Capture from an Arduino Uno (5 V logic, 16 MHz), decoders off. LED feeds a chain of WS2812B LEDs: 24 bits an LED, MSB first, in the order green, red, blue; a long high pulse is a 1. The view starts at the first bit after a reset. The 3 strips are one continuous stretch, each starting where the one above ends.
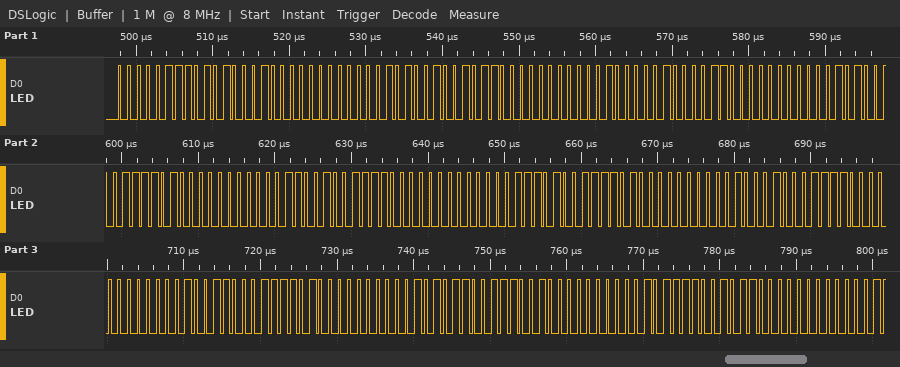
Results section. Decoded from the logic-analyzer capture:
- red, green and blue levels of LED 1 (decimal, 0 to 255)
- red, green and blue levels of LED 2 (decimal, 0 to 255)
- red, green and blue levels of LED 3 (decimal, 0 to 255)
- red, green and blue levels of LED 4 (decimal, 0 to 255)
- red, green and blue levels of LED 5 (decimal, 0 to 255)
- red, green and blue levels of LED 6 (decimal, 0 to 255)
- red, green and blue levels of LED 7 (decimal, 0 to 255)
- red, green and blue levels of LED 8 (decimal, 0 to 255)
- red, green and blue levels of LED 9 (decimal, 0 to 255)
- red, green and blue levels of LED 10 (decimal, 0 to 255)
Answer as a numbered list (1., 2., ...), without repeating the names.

1. 81, 7, 0
2. 75, 10, 0
3. 67, 16, 0
4. 61, 20, 0
5. 60, 25, 0
6. 61, 29, 0
7. 60, 34, 0
8. 61, 38, 0
9. 57, 43, 0
10. 44, 47, 0
